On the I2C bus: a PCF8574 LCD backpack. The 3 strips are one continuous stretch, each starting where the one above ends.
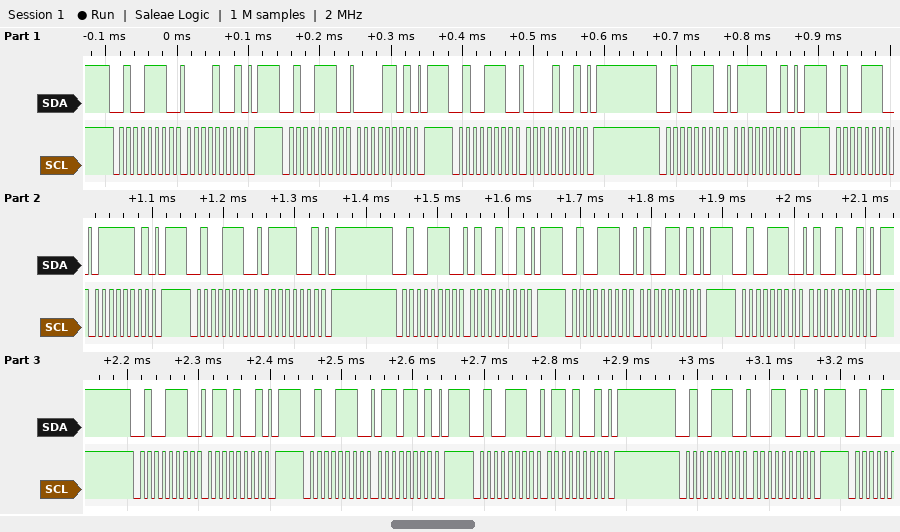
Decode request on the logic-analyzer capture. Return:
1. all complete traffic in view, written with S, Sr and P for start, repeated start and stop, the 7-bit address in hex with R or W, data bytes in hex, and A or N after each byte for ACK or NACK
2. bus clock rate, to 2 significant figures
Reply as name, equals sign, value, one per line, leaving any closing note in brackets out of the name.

all complete traffic in view, written with S, Sr and P for start, repeated start and stop, the 7-bit address in hex with R or W, data bytes in hex, and A or N after each byte for ACK or NACK = S 27W A 09 A P S 27W A 0D A P S 27W A 09 A P S 27W A 79 A P S 27W A 7D A P S 27W A 79 A P S 27W A 49 A P S 27W A 4D A P S 27W A 49 A P S 27W A 69 A P S 27W A 6D A P S 27W A 69 A P S 27W A 19 A P
bus clock rate, to 2 significant figures = 100 kHz
